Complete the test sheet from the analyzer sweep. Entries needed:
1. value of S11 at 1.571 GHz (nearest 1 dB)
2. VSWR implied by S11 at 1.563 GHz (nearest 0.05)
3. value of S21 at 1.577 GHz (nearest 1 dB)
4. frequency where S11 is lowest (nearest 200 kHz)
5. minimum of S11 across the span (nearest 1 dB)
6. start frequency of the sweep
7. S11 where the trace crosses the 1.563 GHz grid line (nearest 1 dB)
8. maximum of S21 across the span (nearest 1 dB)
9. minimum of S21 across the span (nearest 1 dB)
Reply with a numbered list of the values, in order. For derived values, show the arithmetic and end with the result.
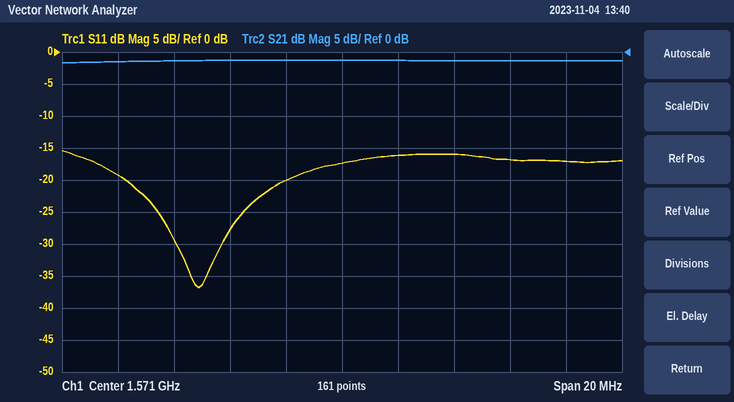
1. -17 dB
2. |Γ| = 10^(-19/20) = 0.1122; VSWR = (1 + 0.1122)/(1 − 0.1122) ≈ 1.25
3. -1 dB
4. 1.5658 GHz
5. -37 dB
6. 1.561 GHz
7. -19 dB
8. -1 dB
9. -2 dB
